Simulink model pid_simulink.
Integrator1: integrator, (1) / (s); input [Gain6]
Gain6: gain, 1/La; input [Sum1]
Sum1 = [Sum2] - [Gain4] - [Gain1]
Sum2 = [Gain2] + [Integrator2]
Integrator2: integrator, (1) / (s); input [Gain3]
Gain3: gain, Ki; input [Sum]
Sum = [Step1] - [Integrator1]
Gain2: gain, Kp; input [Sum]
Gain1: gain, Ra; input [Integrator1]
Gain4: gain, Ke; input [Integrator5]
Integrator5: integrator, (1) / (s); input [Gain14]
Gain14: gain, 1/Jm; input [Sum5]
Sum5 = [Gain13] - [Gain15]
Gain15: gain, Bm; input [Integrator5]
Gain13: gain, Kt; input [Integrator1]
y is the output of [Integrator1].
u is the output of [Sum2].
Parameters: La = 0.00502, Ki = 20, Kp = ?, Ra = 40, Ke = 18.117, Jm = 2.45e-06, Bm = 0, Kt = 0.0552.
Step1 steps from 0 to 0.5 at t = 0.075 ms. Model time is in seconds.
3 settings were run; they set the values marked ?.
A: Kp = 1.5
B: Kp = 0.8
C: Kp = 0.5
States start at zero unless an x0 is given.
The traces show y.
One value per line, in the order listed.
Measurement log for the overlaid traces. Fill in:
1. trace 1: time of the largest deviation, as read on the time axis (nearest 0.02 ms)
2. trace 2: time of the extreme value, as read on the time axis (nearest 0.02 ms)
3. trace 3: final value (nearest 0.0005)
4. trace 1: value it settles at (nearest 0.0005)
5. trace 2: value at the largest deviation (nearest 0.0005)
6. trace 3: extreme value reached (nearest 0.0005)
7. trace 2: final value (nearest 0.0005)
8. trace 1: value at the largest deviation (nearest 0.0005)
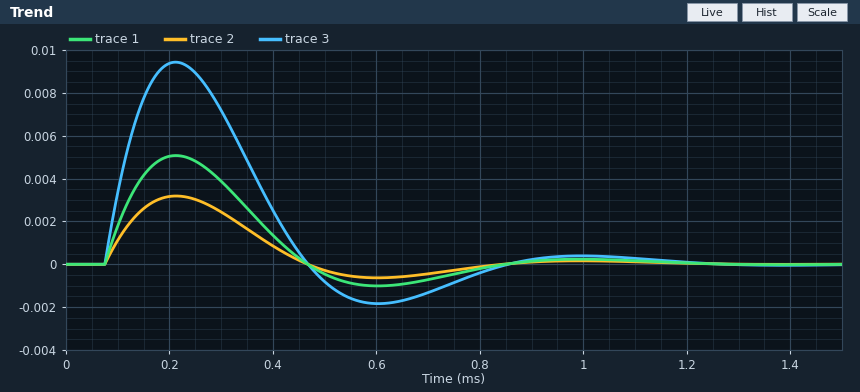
0.22 ms
0.22 ms
0.0000
0.0000
0.0030
0.0095
0.0000
0.0050
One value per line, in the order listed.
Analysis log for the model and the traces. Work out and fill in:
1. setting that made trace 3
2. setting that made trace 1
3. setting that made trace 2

A
B
C
